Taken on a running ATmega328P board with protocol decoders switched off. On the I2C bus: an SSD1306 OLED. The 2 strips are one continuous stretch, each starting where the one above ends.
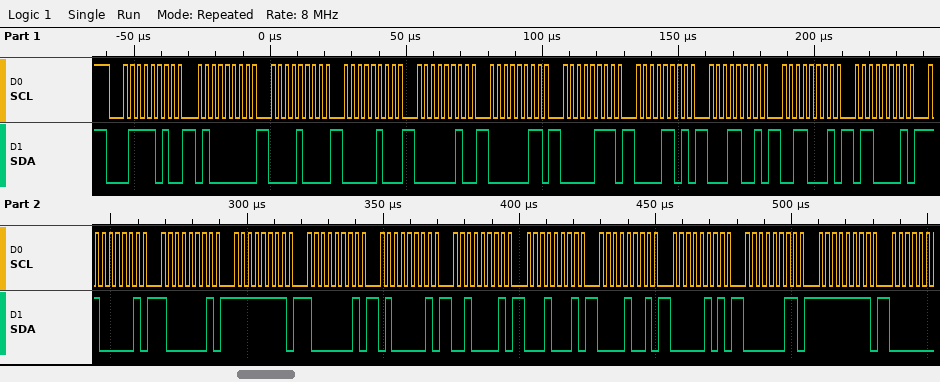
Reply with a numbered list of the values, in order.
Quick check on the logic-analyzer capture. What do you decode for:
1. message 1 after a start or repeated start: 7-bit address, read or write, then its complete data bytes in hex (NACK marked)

1. 0x3D write: 40 08 04 02 03 07 0D 19 31 61 C1 81 FF 81 41 21 11 09 05 03 FF
